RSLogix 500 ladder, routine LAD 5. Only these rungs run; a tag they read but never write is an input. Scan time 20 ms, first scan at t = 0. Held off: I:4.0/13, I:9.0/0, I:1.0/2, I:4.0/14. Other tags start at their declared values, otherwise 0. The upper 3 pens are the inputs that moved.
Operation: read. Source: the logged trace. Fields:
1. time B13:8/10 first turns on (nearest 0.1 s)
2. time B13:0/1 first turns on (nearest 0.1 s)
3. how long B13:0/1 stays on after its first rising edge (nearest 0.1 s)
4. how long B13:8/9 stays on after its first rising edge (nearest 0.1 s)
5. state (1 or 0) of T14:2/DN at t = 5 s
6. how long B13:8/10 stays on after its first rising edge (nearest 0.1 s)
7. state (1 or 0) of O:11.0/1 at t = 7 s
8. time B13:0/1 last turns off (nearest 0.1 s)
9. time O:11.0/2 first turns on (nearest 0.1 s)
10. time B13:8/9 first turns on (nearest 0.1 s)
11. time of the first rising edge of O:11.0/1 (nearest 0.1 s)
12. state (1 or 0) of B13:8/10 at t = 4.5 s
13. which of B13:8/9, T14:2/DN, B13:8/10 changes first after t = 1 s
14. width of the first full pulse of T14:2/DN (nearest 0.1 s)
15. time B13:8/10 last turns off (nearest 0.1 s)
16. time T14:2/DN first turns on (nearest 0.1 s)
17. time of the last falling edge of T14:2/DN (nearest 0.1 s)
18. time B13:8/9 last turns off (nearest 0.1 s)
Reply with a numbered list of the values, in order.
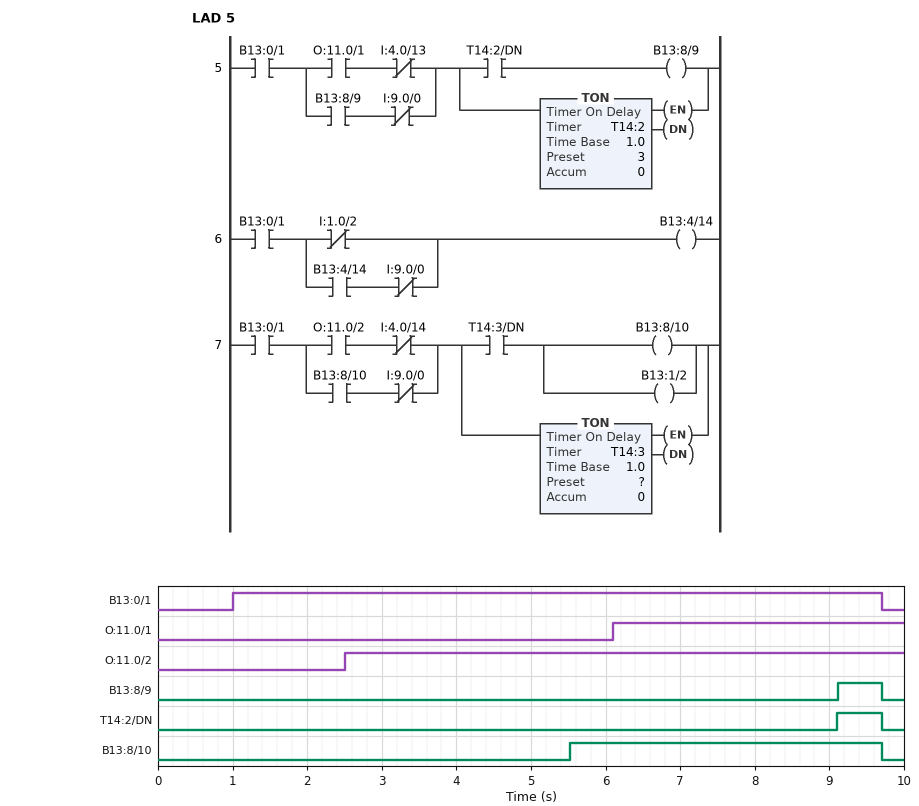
1. 5.5 s
2. 1.0 s
3. 8.7 s
4. 0.6 s
5. 0
6. 4.2 s
7. 1
8. 9.7 s
9. 2.5 s
10. 9.1 s
11. 6.1 s
12. 0
13. B13:8/10
14. 0.6 s
15. 9.7 s
16. 9.1 s
17. 9.7 s
18. 9.7 s
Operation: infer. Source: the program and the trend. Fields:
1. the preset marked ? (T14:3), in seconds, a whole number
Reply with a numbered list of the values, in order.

1. 3 s
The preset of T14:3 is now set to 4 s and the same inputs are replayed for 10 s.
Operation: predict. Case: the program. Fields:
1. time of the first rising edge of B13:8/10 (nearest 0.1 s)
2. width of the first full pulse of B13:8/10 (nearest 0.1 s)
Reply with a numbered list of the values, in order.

1. 6.5 s
2. 3.2 s
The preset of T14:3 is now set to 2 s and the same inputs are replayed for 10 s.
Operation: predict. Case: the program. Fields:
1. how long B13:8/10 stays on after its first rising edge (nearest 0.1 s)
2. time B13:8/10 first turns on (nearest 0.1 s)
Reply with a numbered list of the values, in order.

1. 5.2 s
2. 4.5 s
